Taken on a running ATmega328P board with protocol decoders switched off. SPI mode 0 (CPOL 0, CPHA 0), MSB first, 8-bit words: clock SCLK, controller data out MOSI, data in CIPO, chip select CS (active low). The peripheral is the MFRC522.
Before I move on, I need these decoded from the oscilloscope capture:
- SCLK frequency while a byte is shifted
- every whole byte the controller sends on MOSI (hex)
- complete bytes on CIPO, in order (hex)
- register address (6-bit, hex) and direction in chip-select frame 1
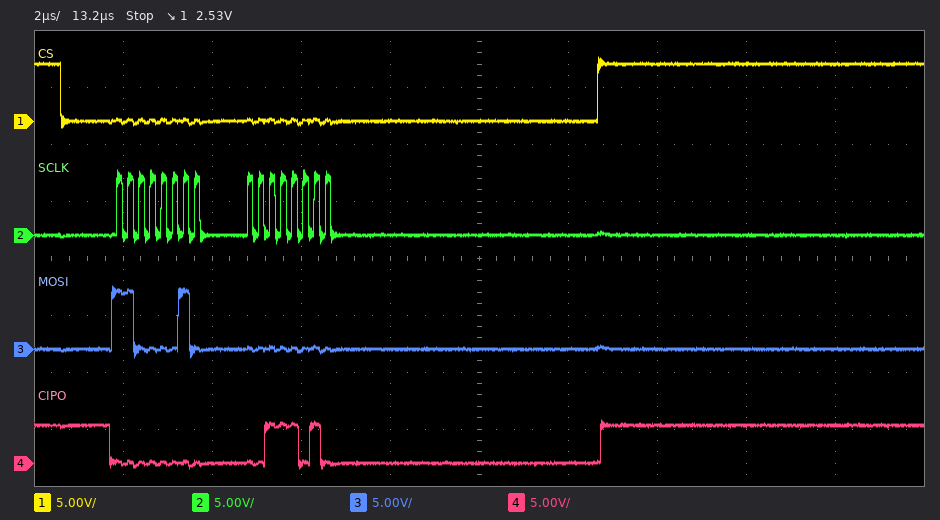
4 MHz
0xC2 0x00
0x00 0x3A
0x21 read
